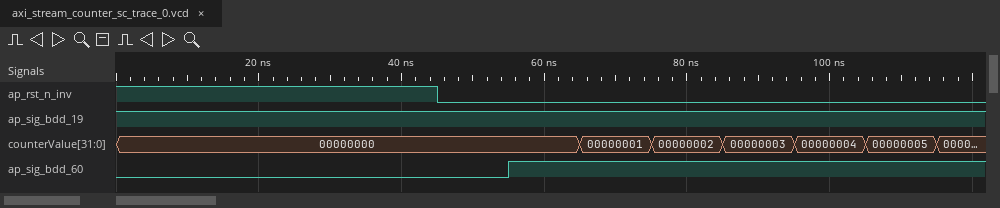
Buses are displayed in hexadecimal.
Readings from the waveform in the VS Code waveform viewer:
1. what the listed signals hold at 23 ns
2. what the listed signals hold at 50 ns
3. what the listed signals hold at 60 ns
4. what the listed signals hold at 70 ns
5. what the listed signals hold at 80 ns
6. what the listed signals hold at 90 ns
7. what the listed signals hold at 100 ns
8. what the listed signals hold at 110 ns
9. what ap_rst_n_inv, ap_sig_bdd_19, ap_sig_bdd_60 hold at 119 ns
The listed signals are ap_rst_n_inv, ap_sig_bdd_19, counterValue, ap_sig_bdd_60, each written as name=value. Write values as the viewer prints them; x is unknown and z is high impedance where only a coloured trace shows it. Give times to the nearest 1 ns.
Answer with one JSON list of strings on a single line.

["ap_rst_n_inv=1, ap_sig_bdd_19=1, counterValue=00000000, ap_sig_bdd_60=0", "ap_rst_n_inv=0, ap_sig_bdd_19=1, counterValue=00000000, ap_sig_bdd_60=0", "ap_rst_n_inv=0, ap_sig_bdd_19=1, counterValue=00000000, ap_sig_bdd_60=1", "ap_rst_n_inv=0, ap_sig_bdd_19=1, counterValue=00000001, ap_sig_bdd_60=1", "ap_rst_n_inv=0, ap_sig_bdd_19=1, counterValue=00000002, ap_sig_bdd_60=1", "ap_rst_n_inv=0, ap_sig_bdd_19=1, counterValue=00000003, ap_sig_bdd_60=1", "ap_rst_n_inv=0, ap_sig_bdd_19=1, counterValue=00000004, ap_sig_bdd_60=1", "ap_rst_n_inv=0, ap_sig_bdd_19=1, counterValue=00000005, ap_sig_bdd_60=1", "ap_rst_n_inv=0, ap_sig_bdd_19=1, ap_sig_bdd_60=1"]
